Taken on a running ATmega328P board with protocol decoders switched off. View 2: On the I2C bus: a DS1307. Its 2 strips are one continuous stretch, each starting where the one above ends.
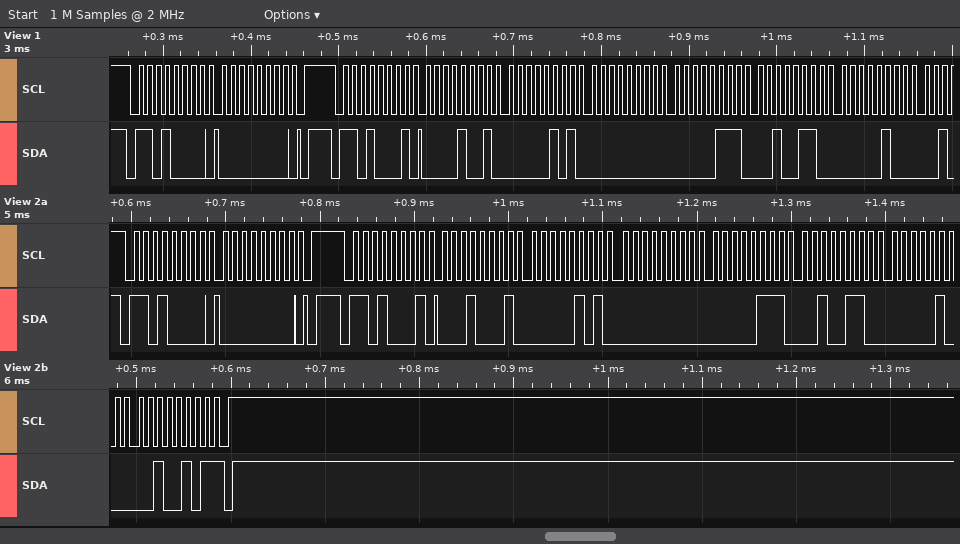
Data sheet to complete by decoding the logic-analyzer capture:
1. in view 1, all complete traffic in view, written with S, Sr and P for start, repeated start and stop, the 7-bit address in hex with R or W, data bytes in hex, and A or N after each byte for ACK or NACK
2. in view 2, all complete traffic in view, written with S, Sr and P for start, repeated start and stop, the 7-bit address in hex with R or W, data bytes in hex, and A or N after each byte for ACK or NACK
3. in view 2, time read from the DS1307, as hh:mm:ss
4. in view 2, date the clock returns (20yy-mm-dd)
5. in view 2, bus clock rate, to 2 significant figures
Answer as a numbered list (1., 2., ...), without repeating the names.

1. S 68W A 00 A P S 68R A 09 A 05 A 00 A 07 A 26 A 04 A
2. S 68W A 00 A P S 68R A 11 A 05 A 00 A 07 A 26 A 04 A 25 N P
3. 00:05:11
4. 2025-04-26
5. 100 kHz
